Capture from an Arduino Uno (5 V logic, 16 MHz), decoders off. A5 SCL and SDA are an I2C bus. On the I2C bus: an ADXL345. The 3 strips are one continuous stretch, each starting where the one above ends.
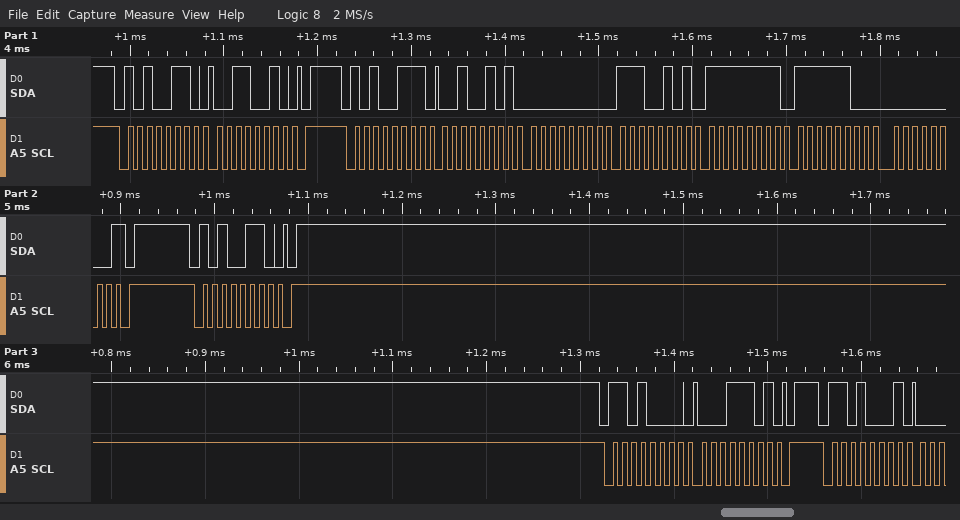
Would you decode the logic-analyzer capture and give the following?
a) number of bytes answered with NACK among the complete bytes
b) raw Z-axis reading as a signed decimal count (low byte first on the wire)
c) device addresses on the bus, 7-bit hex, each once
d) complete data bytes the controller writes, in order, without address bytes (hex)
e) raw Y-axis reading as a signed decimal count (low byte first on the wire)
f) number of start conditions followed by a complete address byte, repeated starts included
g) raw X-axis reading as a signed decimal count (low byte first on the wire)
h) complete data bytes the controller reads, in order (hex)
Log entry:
1
252
0x53 0x68
32 1D
-27
5
37
25 00 E5 FF FC 00
